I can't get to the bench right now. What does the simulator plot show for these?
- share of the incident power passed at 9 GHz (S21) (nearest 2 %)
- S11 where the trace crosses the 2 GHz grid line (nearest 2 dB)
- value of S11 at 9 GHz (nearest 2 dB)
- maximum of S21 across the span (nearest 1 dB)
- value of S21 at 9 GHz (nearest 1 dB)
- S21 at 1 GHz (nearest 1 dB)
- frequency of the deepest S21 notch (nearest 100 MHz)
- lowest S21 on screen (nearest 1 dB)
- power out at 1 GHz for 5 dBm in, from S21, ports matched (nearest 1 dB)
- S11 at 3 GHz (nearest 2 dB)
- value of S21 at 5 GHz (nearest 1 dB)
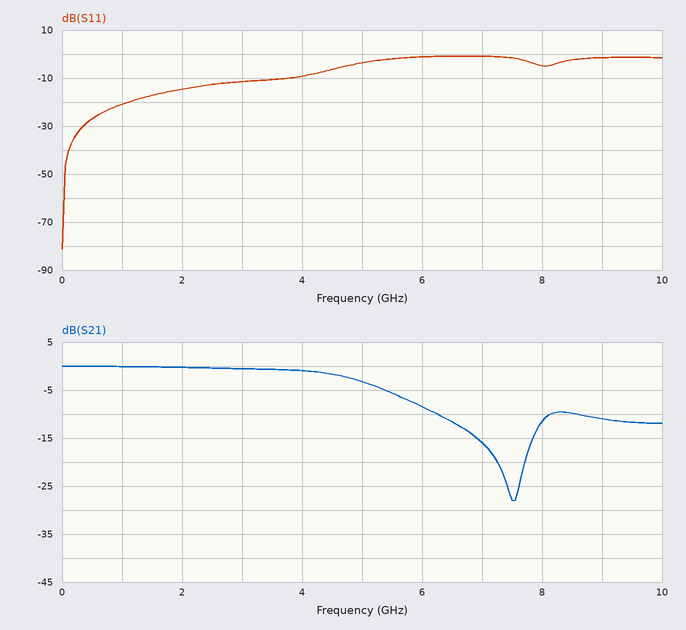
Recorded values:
8 %
-14 dB
-2 dB
0 dB
-11 dB
0 dB
7.5 GHz
-28 dB
5 dBm
-12 dB
-3 dB
